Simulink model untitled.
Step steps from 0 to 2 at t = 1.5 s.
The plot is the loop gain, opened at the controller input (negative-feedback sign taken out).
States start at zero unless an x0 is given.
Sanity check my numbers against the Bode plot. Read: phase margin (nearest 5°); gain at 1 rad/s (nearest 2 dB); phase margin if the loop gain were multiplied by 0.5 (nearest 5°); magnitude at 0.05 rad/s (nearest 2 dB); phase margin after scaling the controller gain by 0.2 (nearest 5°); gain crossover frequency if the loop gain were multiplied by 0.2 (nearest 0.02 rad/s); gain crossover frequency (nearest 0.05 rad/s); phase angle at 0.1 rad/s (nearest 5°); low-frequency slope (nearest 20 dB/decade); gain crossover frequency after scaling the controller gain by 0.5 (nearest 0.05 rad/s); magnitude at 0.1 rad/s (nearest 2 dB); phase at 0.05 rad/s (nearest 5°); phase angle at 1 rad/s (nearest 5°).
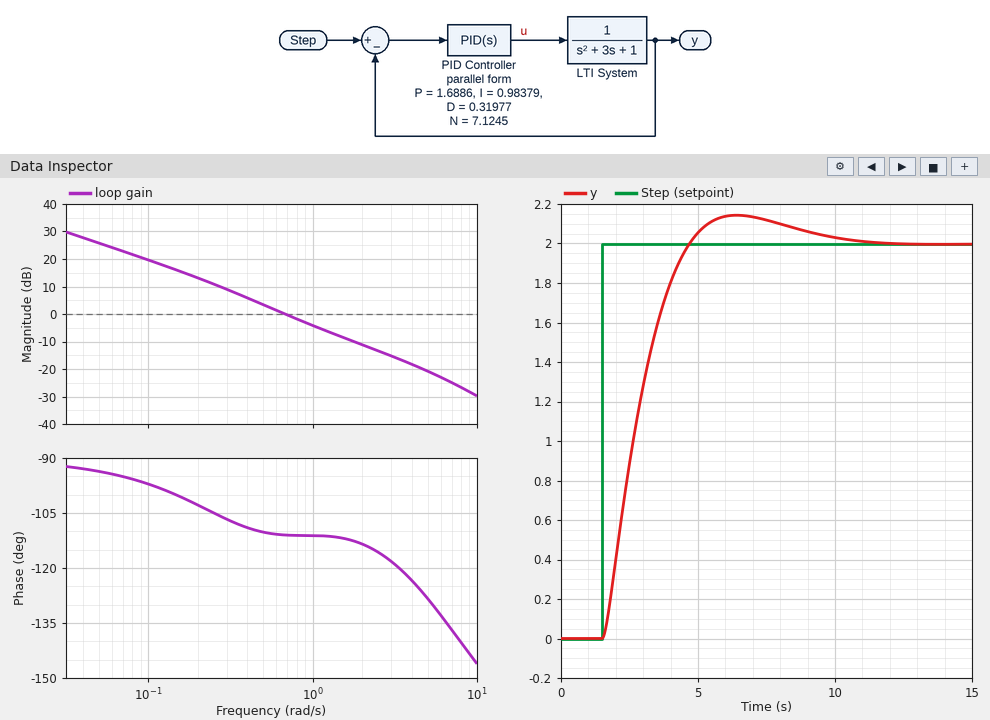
70°
-4 dB
70°
26 dB
80°
0.18 rad/s
0.70 rad/s
-95°
-20 dB/decade
0.40 rad/s
20 dB
-95°
-110°
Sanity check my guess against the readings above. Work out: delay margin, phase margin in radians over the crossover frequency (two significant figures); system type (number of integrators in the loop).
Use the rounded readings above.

1.7 s
1
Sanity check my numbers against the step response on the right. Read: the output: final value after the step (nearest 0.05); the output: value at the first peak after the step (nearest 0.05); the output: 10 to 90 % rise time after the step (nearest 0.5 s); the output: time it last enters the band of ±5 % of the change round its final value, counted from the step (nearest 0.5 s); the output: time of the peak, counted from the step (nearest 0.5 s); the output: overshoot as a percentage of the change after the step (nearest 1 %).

2.00
2.15
2.0 s
6.5 s
5.0 s
7 %
